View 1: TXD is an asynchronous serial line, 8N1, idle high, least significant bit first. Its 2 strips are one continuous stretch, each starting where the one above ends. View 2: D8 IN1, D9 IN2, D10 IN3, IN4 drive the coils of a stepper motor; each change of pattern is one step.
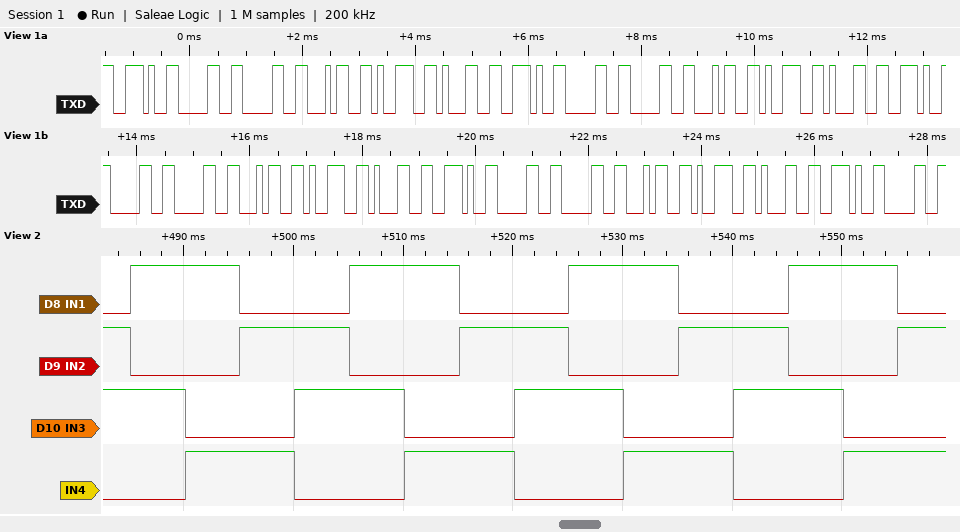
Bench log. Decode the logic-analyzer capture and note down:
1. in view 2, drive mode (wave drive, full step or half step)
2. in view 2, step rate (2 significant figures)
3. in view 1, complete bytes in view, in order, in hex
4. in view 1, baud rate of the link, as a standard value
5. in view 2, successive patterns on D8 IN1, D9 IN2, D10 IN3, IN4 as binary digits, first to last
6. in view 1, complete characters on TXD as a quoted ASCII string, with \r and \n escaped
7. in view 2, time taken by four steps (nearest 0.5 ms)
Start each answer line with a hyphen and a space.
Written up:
- full step
- 200 steps/s
- 2E 30 30 34 39 31 2E 30 30 34 39 31 2E 30 30 34 39 31 2E 30 30 34 39 31 2E 30
- 9600 baud
- 0110 1010 1001 0101 0110 1010 1001 0101 0110 1010 1001 0101 0110 1010 1001 0101
- ".00491.00491.00491.00491.0"
- 20.0 ms
